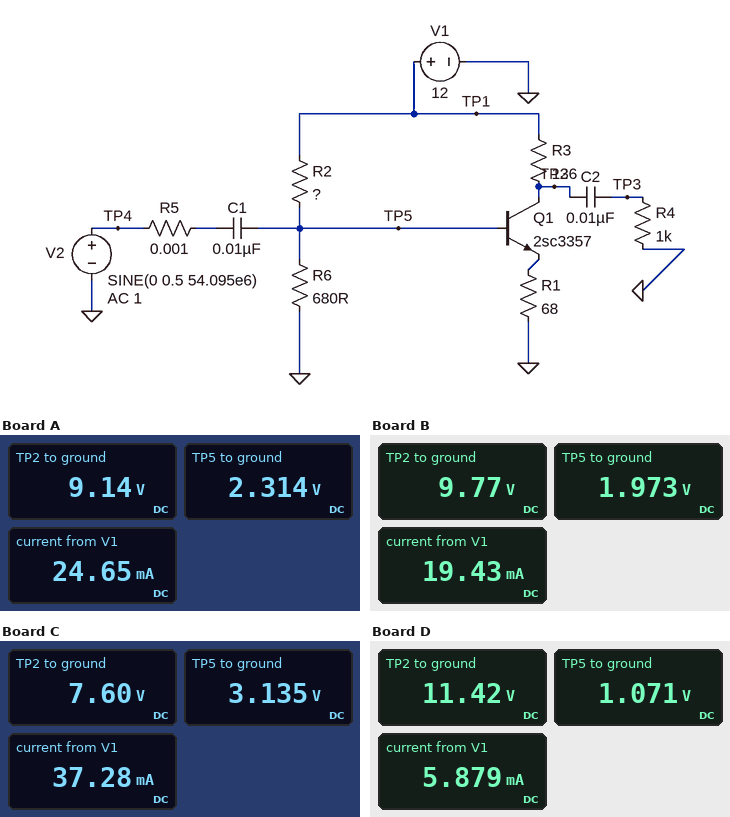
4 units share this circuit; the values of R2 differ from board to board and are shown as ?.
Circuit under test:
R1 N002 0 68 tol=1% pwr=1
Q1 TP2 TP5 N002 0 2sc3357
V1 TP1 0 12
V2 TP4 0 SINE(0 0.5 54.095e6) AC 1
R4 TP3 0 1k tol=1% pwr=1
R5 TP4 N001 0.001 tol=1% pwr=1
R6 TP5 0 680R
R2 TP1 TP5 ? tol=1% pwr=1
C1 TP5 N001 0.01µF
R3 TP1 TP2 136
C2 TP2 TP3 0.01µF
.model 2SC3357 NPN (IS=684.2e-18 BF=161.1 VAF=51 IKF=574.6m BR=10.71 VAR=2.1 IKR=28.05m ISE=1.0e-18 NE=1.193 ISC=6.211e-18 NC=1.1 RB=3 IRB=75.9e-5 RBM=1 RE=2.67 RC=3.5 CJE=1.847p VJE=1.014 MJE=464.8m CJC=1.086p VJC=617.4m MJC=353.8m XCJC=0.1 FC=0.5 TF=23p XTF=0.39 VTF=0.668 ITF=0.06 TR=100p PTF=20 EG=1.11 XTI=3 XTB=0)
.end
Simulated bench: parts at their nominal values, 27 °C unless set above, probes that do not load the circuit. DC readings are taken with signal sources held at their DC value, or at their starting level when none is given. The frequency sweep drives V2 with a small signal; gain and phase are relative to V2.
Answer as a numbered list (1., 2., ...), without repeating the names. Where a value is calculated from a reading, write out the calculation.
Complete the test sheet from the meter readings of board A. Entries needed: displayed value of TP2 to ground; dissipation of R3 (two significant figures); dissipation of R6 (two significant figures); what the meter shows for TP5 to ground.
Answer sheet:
1. 9.14 V
2. (12 V - 9.14 V)^2 / 136 Ω = 60 mW
3. (2.314 V)^2 / 680 Ω = 7.9 mW
4. 2.314 V
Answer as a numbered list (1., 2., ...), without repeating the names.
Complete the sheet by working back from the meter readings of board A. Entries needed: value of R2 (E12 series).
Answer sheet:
1. 2.7 kΩ
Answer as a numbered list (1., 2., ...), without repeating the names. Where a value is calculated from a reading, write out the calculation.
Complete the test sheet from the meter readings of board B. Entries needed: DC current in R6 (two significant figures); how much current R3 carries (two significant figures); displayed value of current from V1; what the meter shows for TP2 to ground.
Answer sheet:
1. (1.973 V) / 680 Ω = 2.9 mA
2. (12 V - 9.77 V) / 136 Ω = 16 mA
3. 19.43 mA
4. 9.77 V
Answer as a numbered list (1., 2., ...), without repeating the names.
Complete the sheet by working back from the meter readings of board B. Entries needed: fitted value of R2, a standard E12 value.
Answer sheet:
1. 3.3 kΩ
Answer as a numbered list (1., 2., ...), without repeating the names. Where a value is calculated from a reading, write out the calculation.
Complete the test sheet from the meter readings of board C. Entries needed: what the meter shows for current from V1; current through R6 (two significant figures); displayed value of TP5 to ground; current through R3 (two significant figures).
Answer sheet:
1. 37.28 mA
2. (3.135 V) / 680 Ω = 4.6 mA
3. 3.135 V
4. (12 V - 7.6 V) / 136 Ω = 32 mA
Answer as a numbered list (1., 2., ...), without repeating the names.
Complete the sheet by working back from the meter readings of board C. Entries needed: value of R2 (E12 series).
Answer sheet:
1. 1.8 kΩ
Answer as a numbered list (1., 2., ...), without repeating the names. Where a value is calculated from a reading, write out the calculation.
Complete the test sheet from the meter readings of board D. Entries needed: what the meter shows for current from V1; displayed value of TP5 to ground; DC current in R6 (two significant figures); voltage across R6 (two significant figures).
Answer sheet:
1. 5.879 mA
2. 1.071 V
3. (1.071 V) / 680 Ω = 1.6 mA
4. 1.071 V = 1.1 V
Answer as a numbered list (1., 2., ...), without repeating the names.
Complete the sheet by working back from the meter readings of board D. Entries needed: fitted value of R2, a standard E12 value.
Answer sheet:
1. 6.8 kΩ
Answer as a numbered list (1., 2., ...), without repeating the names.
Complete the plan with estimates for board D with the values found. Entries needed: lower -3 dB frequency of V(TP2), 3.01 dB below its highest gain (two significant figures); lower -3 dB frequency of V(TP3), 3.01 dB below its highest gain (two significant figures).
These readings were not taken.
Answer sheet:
1. 26 kHz
2. 33 kHz
